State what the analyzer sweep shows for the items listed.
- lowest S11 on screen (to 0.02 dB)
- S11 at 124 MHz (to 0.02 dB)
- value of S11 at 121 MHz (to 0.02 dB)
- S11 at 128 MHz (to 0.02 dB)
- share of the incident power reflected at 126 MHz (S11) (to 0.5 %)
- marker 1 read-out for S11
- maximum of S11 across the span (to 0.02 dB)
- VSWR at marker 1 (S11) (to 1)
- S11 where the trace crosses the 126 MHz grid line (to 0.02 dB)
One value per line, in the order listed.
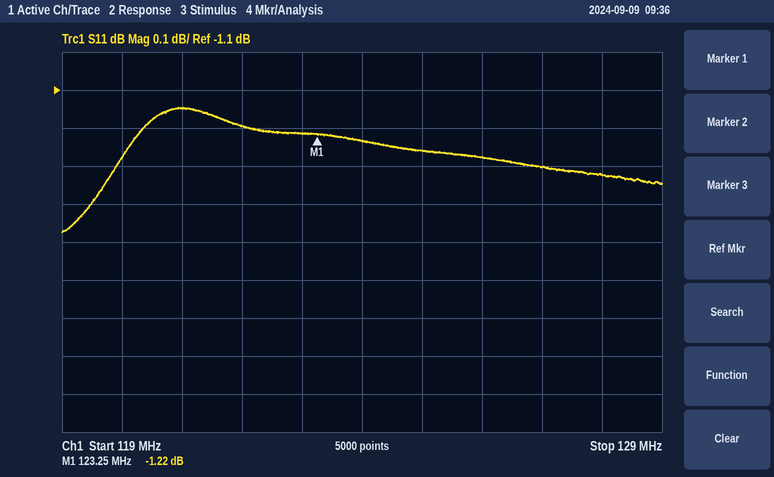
-1.48 dB
-1.24 dB
-1.14 dB
-1.32 dB
74.5 %
-1.22 dB
-1.14 dB
14
-1.28 dB
